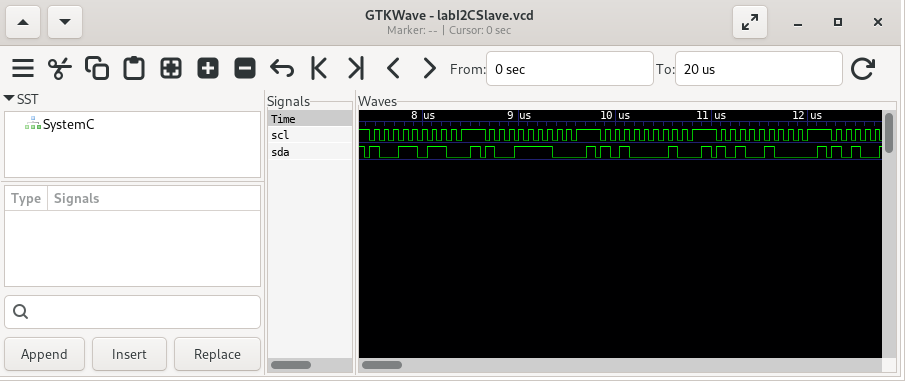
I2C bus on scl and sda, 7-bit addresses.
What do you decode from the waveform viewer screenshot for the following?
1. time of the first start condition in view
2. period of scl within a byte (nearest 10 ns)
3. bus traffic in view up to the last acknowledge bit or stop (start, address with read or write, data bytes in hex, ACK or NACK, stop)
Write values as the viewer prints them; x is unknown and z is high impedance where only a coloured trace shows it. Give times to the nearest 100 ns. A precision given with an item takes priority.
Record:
7400 ns
100 ns
start, address 4D read ACK, stop, start, address 4F write ACK, stop, start, address 50 read ACK, stop, start, address 52 write ACK, stop
